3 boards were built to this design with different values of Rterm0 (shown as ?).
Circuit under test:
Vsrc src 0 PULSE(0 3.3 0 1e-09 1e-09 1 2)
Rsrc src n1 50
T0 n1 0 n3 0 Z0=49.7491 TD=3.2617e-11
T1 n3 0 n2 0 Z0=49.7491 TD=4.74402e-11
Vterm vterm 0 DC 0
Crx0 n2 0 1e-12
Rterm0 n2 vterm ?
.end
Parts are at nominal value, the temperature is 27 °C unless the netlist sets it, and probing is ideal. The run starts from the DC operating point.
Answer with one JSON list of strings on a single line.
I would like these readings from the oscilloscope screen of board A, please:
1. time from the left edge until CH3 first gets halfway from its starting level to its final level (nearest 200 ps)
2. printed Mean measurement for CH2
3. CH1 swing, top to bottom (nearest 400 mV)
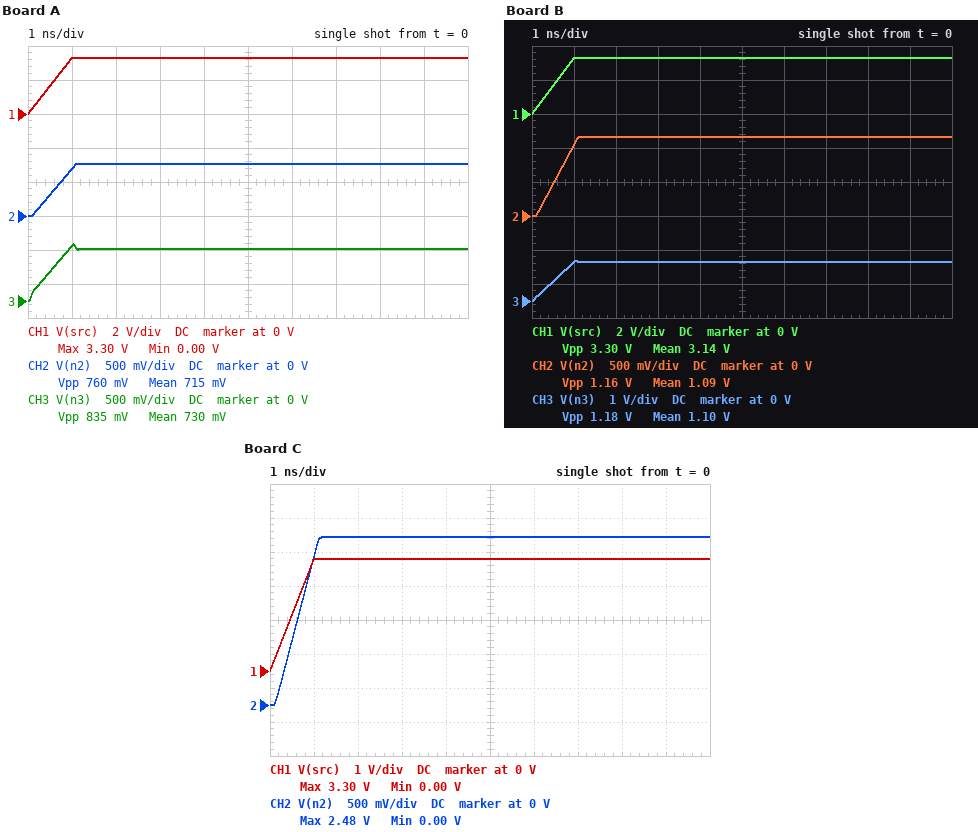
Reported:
["400 ps", "715 mV", "3.2 V"]
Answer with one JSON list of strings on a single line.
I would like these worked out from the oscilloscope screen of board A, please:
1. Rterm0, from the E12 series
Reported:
["15 Ω"]
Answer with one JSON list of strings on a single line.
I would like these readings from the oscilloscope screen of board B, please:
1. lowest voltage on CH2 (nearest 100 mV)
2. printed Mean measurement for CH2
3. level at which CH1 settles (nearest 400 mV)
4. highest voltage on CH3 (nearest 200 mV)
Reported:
["0 V", "1.09 V", "3.2 V", "1.2 V"]
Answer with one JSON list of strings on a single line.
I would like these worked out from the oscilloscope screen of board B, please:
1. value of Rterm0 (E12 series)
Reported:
["27 Ω"]
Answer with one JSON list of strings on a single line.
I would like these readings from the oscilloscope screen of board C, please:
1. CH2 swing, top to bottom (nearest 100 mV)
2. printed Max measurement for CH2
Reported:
["2.5 V", "2.48 V"]
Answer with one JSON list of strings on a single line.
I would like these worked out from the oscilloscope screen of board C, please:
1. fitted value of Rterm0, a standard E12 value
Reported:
["150 Ω"]
